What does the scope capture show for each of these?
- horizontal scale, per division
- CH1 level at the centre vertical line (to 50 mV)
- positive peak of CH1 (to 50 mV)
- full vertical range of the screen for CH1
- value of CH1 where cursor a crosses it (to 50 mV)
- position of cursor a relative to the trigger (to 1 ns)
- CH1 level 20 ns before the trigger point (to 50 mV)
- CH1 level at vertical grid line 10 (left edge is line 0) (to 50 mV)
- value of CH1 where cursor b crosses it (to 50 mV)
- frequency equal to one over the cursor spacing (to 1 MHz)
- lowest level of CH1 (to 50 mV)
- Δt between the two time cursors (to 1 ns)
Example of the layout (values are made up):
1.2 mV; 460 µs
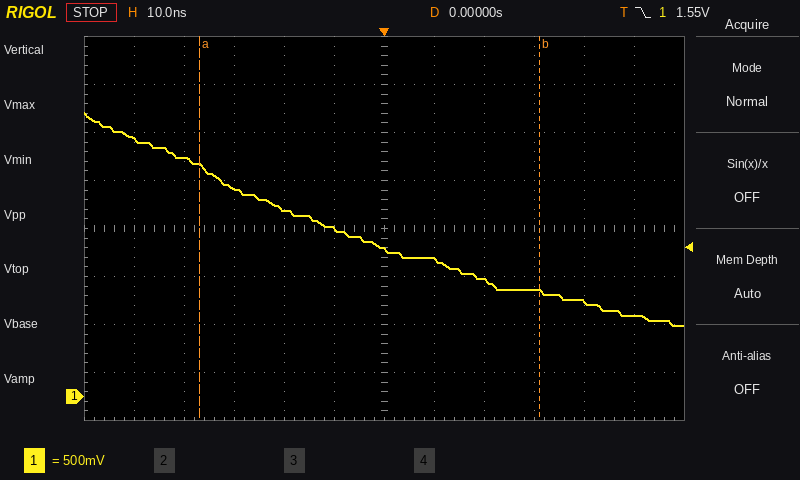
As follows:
10 ns; 1.55 V; 2.95 V; 4 V; 2.40 V; -37 ns; 1.95 V; 1.00 V; 1.10 V; 15 MHz; 750 mV; 68 ns
